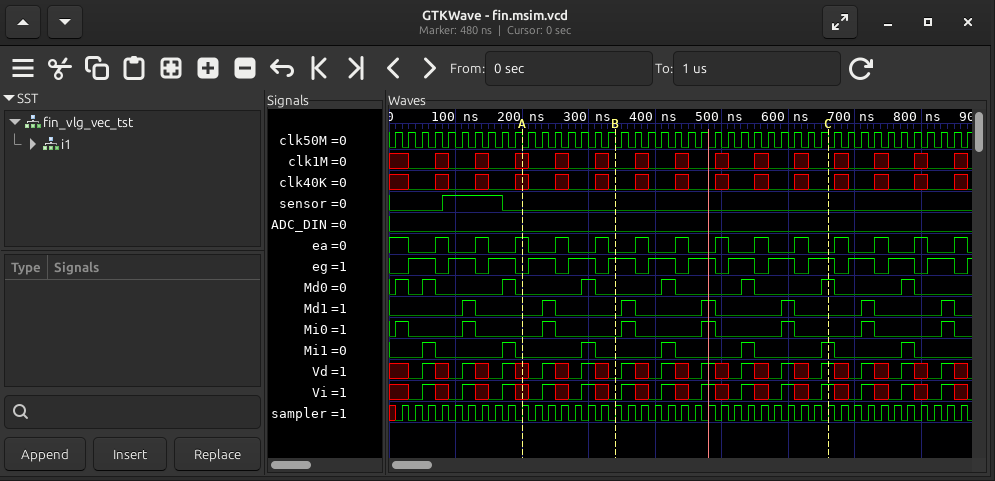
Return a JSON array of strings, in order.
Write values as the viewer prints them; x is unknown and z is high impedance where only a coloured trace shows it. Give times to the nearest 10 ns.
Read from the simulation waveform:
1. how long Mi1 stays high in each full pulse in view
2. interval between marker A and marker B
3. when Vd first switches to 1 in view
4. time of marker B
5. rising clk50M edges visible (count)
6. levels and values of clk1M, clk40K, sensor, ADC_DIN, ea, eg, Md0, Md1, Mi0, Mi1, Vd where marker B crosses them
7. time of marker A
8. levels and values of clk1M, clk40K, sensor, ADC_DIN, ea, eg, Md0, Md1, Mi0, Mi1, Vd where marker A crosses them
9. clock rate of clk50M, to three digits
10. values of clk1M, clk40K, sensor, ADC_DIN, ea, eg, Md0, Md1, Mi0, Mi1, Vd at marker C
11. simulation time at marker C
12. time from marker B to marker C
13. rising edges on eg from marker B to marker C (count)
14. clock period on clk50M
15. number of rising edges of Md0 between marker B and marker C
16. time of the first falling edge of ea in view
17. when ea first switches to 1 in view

["20 ns, 20 ns, 20 ns, 20 ns, 20 ns, 20 ns, 20 ns", "140 ns", "50 ns", "340 ns", "44", "clk1M=0, clk40K=0, sensor=0, ADC_DIN=0, ea=0, eg=1, Md0=0, Md1=0, Mi0=0, Mi1=0, Vd=0", "200 ns", "clk1M=x, clk40K=x, sensor=0, ADC_DIN=0, ea=1, eg=0, Md0=0, Md1=0, Mi0=0, Mi1=0, Vd=x", "50.0 MHz", "clk1M=0, clk40K=0, sensor=0, ADC_DIN=0, ea=0, eg=1, Md0=1, Md1=0, Mi0=0, Mi1=1, Vd=1", "660 ns", "320 ns", "5", "20 ns", "3", "30 ns", "70 ns"]
